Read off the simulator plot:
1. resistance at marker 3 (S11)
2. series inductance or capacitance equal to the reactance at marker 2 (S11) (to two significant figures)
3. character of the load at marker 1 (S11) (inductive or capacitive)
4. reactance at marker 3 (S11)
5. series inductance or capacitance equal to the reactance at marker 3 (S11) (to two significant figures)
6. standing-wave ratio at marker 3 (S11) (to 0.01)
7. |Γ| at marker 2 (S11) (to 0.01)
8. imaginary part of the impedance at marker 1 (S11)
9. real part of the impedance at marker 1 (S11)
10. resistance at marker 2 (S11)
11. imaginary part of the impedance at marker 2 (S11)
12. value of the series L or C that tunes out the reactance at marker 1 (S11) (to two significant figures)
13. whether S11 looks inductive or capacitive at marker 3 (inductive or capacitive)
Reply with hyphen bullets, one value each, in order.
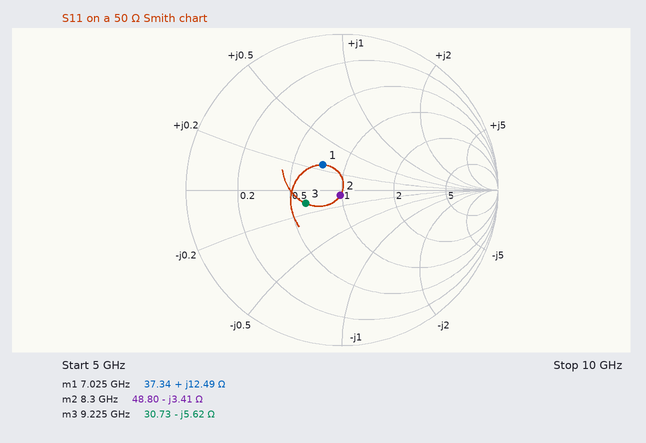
- 30.73 Ω
- 5.6 pF
- inductive
- -5.62 Ω
- 3.1 pF
- 1.66
- 0.04
- +12.49 Ω
- 37.34 Ω
- 48.80 Ω
- -3.41 Ω
- 1.8 pF
- capacitive
